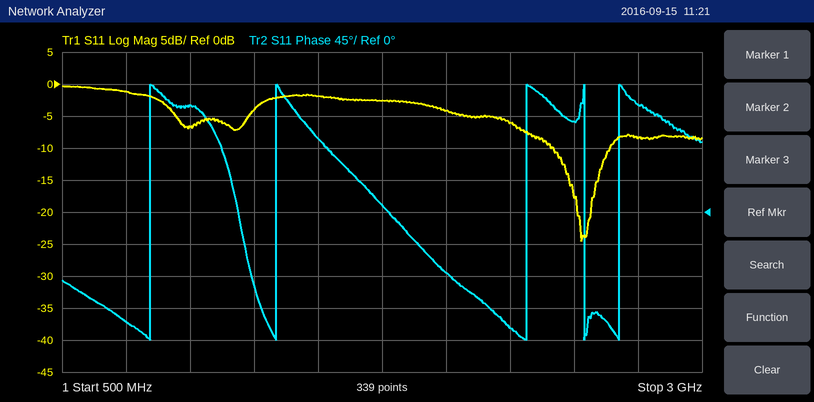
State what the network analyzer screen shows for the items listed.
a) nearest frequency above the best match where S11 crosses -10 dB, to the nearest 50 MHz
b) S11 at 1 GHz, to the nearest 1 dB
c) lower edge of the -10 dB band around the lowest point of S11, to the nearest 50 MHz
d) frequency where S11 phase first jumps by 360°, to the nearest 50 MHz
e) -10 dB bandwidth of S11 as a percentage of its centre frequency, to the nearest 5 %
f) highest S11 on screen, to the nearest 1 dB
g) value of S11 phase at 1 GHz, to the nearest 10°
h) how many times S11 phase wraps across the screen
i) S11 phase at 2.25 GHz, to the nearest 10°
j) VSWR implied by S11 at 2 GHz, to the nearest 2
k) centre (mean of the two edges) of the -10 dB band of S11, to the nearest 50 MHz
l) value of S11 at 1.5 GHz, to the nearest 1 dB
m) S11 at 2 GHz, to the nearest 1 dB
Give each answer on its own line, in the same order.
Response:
2.65 GHz
-7 dB
2.40 GHz
850 MHz
10 %
0 dB
150°
5
-160°
4
2.55 GHz
-2 dB
-4 dB
